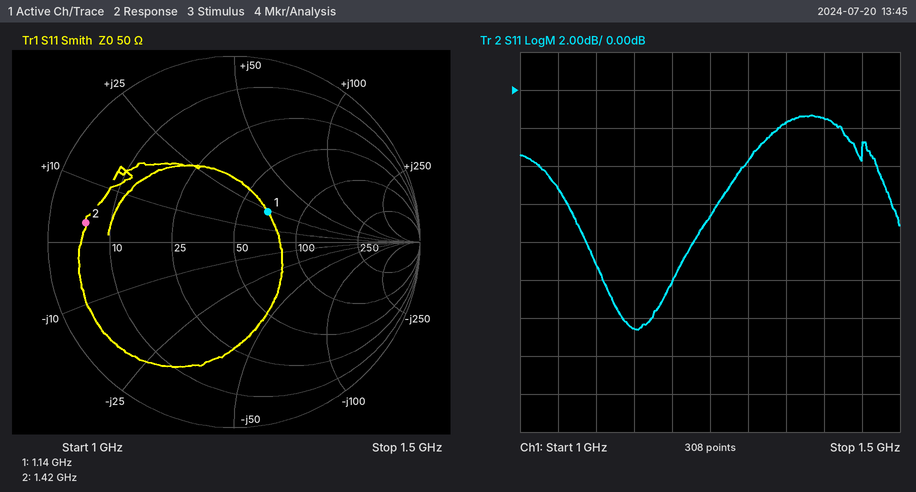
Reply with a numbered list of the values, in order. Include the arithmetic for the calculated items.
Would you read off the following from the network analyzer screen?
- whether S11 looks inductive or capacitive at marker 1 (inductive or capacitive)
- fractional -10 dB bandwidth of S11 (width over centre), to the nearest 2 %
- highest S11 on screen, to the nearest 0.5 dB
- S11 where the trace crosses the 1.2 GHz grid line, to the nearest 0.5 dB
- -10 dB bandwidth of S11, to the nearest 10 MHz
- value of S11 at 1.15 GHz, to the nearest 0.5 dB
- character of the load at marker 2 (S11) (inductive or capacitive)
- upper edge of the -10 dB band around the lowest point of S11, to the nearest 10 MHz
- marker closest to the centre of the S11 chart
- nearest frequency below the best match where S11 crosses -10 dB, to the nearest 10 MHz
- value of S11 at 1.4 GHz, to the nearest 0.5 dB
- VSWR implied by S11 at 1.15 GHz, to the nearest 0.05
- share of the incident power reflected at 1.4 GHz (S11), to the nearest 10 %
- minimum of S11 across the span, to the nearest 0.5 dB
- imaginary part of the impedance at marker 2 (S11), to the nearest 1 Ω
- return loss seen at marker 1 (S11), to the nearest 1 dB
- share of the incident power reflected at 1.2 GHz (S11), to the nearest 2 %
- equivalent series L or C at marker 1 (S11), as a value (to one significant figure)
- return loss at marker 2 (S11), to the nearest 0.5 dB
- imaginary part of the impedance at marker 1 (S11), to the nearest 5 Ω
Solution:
1. inductive
2. 90 MHz / 1.155 GHz ≈ 8 %
3. -1.5 dB
4. -10.0 dB
5. 1.20 GHz − 1.11 GHz = 90 MHz
6. -12.5 dB
7. inductive
8. 1.20 GHz
9. marker 1
10. 1.11 GHz
11. -1.5 dB
12. |Γ| = 10^(-12.5/20) = 0.2371; VSWR = (1 + 0.2371)/(1 − 0.2371) ≈ 1.62, so 1.60 to the nearest 0.05
13. 10^(-1.5/10) ≈ 70.8 %, so 70 % to the nearest 10 %
14. -12.5 dB
15. +3 Ω
16. 12 dB
17. 10^(-10/10) ≈ 10 %
18. L = 25 Ω/(2π × 1.14 GHz) ≈ 3 nH
19. 2.0 dB
20. +25 Ω
